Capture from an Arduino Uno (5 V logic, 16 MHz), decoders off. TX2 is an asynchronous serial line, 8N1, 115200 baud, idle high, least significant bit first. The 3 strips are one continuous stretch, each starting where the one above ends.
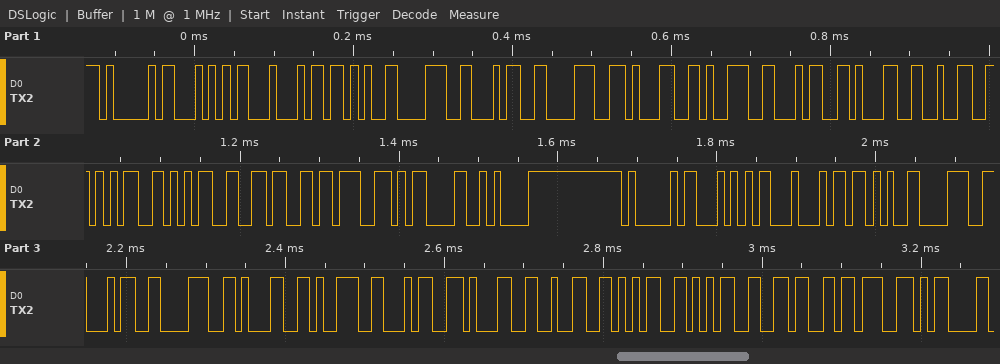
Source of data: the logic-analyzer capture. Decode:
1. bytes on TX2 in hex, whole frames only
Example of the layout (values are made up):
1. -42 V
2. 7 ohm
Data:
1. 41 54 44 2B 38 34 38 31 39 34 31 32 35 35 36 3B 0D 0A 41 54 44 2B 38 34 38 31 39 34 31 32 35 35 36 3B 0D
